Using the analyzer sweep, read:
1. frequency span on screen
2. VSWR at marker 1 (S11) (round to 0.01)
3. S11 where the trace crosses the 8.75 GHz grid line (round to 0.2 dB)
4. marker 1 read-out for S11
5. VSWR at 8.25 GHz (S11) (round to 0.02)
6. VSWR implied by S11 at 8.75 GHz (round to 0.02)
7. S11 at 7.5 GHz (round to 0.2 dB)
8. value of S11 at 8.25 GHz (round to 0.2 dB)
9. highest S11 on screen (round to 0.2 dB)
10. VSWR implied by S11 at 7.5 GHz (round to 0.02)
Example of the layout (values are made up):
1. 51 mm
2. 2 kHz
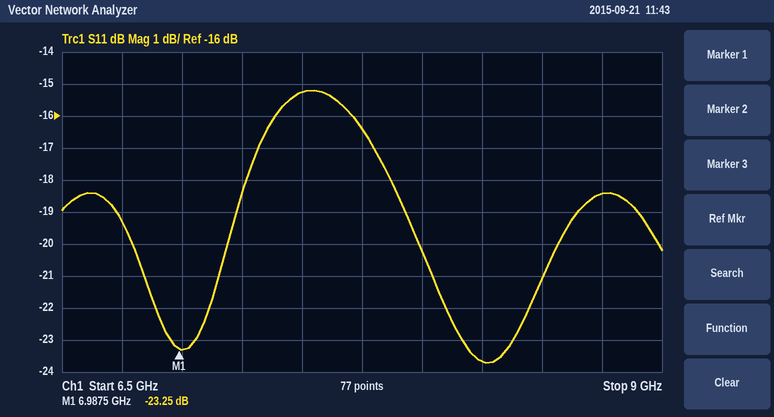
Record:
1. 2.5 GHz
2. 1.15
3. -18.4 dB
4. -23.25 dB
5. 1.14
6. 1.28
7. -15.2 dB
8. -23.6 dB
9. -15.2 dB
10. 1.42
